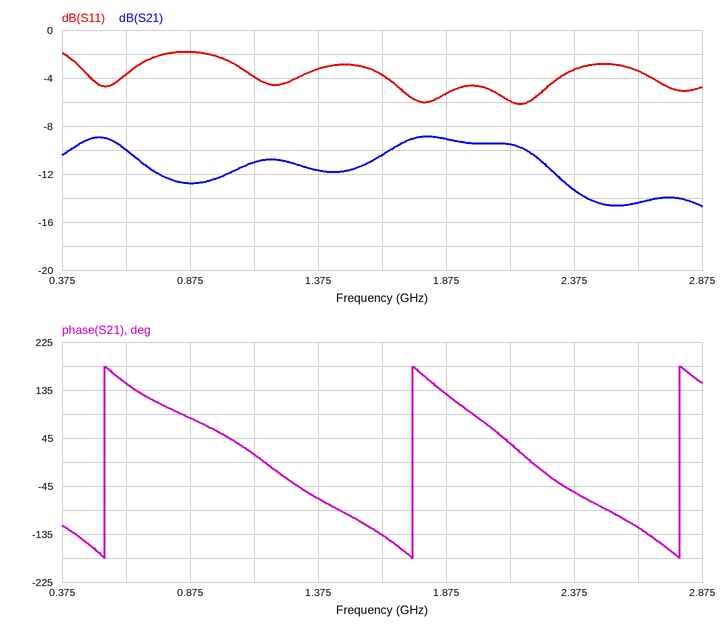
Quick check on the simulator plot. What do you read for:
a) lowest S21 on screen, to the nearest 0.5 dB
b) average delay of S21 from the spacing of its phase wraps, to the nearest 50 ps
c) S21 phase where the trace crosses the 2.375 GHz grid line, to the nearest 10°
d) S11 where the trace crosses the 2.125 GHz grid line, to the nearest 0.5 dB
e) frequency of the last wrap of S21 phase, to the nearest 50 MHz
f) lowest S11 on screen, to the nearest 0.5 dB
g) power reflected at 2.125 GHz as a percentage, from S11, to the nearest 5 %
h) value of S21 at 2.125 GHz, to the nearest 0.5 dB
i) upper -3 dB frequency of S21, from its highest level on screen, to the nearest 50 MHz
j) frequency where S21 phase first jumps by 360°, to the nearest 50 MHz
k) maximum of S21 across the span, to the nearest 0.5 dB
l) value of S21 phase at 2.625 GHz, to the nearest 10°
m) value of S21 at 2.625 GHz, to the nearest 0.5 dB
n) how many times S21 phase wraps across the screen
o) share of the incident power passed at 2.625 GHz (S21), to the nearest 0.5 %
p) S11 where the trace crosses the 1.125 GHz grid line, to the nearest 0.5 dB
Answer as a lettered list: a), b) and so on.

a) -14.5 dB
b) 900 ps
c) -60°
d) -6.0 dB
e) 2.80 GHz
f) -6.0 dB
g) 25 %
h) -9.5 dB
i) 2.30 GHz
j) 550 MHz
k) -9.0 dB
l) -120°
m) -14.5 dB
n) 3
o) 3.5 %
p) -4.0 dB
